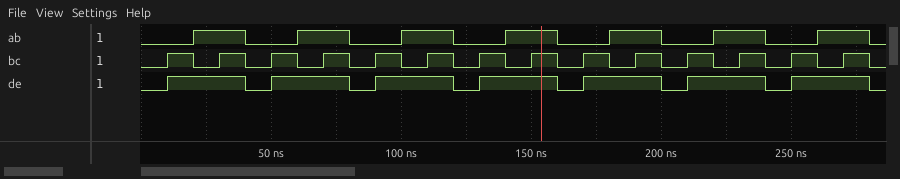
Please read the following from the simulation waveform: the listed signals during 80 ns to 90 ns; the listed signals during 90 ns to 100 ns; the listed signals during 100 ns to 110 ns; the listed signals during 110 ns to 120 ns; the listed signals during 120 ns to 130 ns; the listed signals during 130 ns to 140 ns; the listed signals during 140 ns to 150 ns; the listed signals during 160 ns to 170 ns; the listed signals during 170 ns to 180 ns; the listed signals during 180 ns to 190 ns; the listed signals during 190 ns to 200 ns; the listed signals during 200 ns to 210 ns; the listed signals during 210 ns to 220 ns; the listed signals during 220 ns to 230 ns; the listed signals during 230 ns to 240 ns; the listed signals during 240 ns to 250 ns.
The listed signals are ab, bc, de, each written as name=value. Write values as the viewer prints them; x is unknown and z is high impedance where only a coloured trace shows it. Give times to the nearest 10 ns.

ab=0, bc=0, de=0
ab=0, bc=1, de=1
ab=1, bc=0, de=1
ab=1, bc=1, de=1
ab=0, bc=0, de=0
ab=0, bc=1, de=1
ab=1, bc=0, de=1
ab=0, bc=0, de=0
ab=0, bc=1, de=1
ab=1, bc=0, de=1
ab=1, bc=1, de=1
ab=0, bc=0, de=0
ab=0, bc=1, de=1
ab=1, bc=0, de=1
ab=1, bc=1, de=1
ab=0, bc=0, de=0
